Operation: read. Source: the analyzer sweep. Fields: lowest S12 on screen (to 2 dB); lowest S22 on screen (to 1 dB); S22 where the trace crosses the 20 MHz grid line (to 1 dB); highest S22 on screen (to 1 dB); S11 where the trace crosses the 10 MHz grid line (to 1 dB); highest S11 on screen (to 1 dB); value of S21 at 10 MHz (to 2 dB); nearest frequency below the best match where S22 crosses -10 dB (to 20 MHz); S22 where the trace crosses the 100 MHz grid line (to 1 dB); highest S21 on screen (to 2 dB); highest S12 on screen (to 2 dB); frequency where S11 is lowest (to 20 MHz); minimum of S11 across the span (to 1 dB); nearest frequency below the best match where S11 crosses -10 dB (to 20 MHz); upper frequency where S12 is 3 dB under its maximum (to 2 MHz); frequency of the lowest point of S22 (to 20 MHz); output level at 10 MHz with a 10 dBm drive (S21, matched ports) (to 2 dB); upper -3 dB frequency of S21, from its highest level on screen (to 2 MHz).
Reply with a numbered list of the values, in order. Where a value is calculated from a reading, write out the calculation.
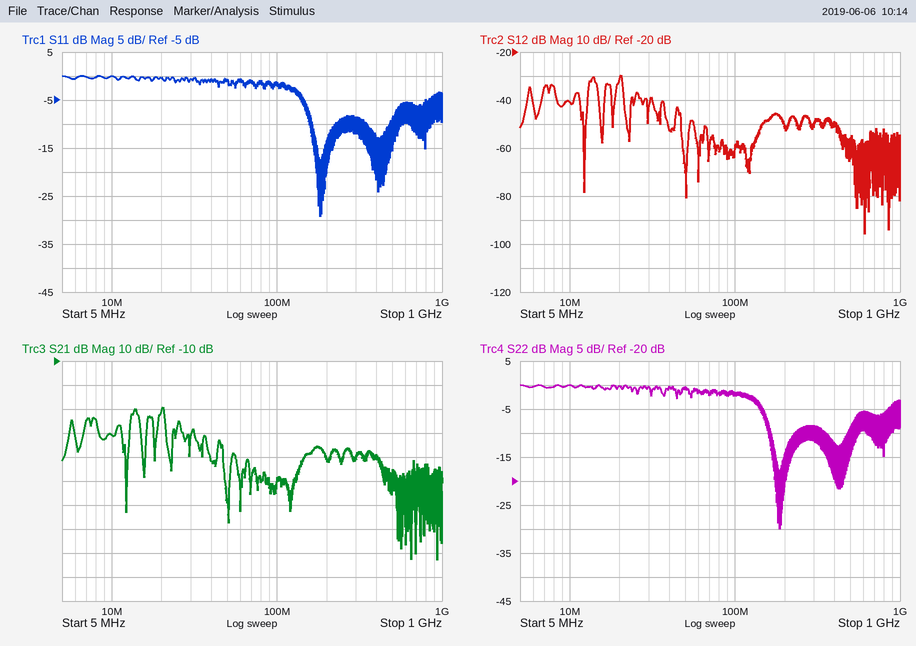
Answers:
1. -96 dB
2. -30 dB
3. 0 dB
4. 0 dB
5. 0 dB
6. 0 dB
7. -40 dB
8. 160 MHz
9. -2 dB
10. -30 dB
11. -30 dB
12. 180 MHz
13. -29 dB
14. 160 MHz
15. 20 MHz
16. 180 MHz
17. 10 dBm + (-40 dB) = -30 dBm
18. 20 MHz
